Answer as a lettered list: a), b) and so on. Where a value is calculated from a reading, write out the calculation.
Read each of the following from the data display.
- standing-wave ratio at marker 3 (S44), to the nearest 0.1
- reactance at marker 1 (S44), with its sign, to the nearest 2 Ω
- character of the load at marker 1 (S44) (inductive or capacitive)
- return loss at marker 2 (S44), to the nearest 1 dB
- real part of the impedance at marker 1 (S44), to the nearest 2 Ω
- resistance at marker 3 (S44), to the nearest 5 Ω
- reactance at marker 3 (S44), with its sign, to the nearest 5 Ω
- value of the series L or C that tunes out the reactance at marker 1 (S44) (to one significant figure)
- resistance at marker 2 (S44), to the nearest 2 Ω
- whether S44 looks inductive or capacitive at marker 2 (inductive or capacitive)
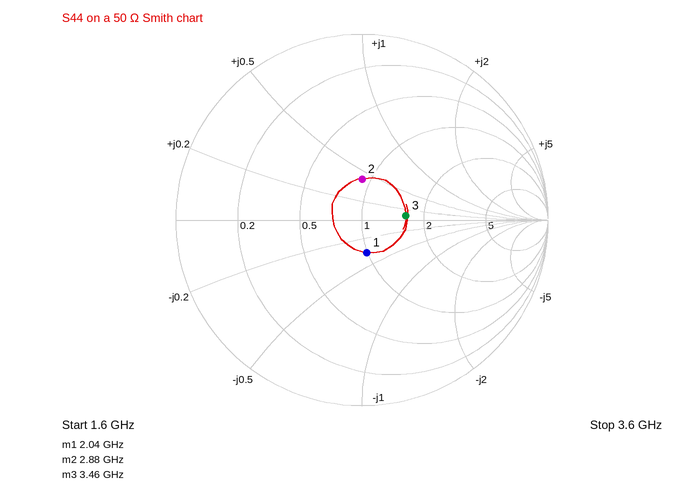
a) 1.6
b) -18 Ω
c) capacitive
d) 13 dB
e) 50 Ω
f) 80 Ω
g) +5 Ω
h) L = 18 Ω/(2π × 2.04 GHz) ≈ 1 nH
i) 46 Ω
j) inductive
